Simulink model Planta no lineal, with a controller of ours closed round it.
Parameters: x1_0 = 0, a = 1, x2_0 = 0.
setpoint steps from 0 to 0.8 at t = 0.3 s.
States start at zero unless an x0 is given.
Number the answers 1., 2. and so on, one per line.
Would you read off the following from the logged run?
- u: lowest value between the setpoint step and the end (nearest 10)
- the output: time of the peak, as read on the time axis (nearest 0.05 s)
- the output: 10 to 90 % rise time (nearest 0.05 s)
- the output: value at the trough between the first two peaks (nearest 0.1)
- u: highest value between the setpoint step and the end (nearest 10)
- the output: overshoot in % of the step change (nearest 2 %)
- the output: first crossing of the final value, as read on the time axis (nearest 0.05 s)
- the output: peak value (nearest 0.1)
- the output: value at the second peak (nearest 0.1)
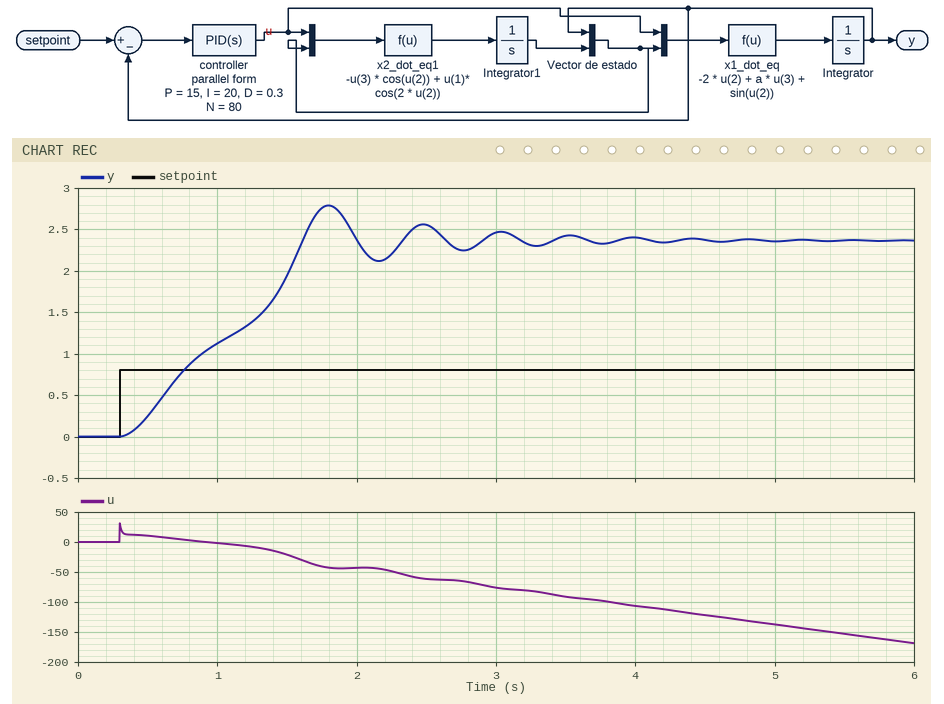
1. -170
2. 1.80 s
3. 1.05 s
4. 2.1
5. 30
6. 18 %
7. 1.60 s
8. 2.8
9. 2.6
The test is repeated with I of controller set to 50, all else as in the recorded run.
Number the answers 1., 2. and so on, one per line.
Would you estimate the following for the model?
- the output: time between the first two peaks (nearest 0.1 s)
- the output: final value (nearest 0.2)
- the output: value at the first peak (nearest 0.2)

1. 0.5 s
2. 2.4
3. 2.8
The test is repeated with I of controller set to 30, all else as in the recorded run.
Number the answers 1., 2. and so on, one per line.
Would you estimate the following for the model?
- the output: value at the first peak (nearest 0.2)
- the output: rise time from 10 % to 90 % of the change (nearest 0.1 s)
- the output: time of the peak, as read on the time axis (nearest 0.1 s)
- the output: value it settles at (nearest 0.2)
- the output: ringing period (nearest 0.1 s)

1. 2.8
2. 1.0 s
3. 1.7 s
4. 2.4
5. 0.6 s
